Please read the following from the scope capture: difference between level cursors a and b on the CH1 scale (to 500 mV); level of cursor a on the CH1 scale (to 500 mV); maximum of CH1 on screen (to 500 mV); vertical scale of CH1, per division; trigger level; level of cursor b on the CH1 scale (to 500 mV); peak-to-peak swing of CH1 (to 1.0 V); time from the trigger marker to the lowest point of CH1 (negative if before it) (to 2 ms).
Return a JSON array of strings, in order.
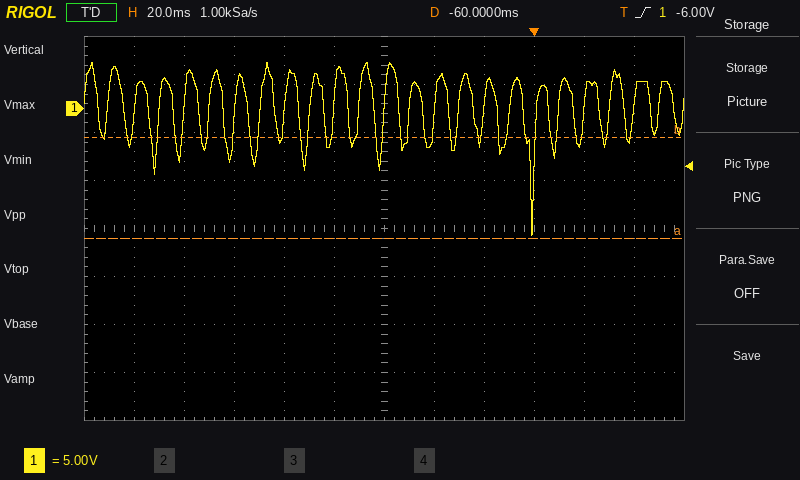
["10.5 V", "-13.5 V", "5.0 V", "5 V", "-6.00 V", "-3.0 V", "18.0 V", "0 ms"]
